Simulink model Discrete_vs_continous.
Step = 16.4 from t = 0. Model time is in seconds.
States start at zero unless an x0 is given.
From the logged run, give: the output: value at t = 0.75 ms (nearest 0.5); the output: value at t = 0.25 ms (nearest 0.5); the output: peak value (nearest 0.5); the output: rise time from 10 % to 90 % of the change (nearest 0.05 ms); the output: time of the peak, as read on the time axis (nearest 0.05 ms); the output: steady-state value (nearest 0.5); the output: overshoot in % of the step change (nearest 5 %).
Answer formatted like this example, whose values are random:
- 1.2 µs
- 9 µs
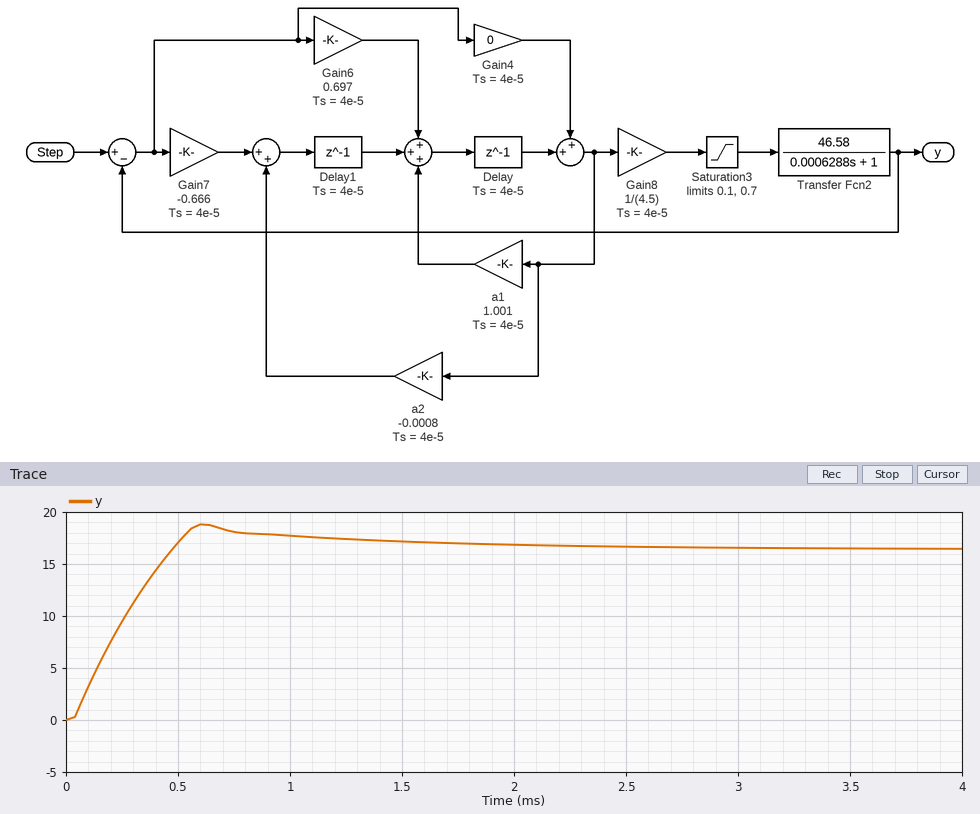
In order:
- 18.0
- 9.5
- 19.0
- 0.35 ms
- 0.60 ms
- 16.5
- 15 %
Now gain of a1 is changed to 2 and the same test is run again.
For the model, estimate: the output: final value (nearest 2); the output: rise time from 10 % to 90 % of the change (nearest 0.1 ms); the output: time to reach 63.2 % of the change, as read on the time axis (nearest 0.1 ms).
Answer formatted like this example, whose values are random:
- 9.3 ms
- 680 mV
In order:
- 32
- 1.4 ms
- 0.7 ms
